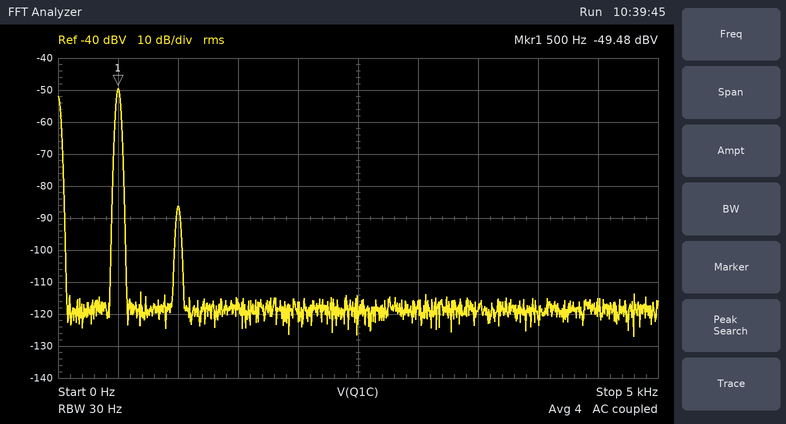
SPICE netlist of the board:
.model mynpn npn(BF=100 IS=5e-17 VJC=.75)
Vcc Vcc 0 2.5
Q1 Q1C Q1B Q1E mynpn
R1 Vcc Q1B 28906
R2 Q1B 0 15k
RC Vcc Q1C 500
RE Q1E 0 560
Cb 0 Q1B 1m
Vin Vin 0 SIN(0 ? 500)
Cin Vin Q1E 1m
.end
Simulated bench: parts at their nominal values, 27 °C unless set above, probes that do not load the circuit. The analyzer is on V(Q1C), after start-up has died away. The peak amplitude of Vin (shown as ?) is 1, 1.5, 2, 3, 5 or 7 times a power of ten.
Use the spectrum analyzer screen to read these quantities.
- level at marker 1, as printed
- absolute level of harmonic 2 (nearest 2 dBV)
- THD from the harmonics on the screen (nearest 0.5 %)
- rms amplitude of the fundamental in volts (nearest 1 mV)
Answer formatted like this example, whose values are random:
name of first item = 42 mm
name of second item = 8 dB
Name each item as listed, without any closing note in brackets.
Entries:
level at marker 1, as printed = -49.48 dBV
absolute level of harmonic 2 = -86 dBV
THD from the harmonics on the screen = 1.5 %
rms amplitude of the fundamental in volts = 3 mV
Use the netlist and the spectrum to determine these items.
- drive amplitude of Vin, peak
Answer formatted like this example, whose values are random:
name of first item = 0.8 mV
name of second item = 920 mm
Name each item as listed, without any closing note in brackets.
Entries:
drive amplitude of Vin, peak = 1.5 mV
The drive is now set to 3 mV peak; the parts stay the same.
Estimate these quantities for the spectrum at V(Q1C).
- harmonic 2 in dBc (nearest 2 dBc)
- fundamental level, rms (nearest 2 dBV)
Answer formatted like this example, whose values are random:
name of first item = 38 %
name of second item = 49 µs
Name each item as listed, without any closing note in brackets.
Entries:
harmonic 2 in dBc = -30 dBc
fundamental level, rms = -44 dBV
